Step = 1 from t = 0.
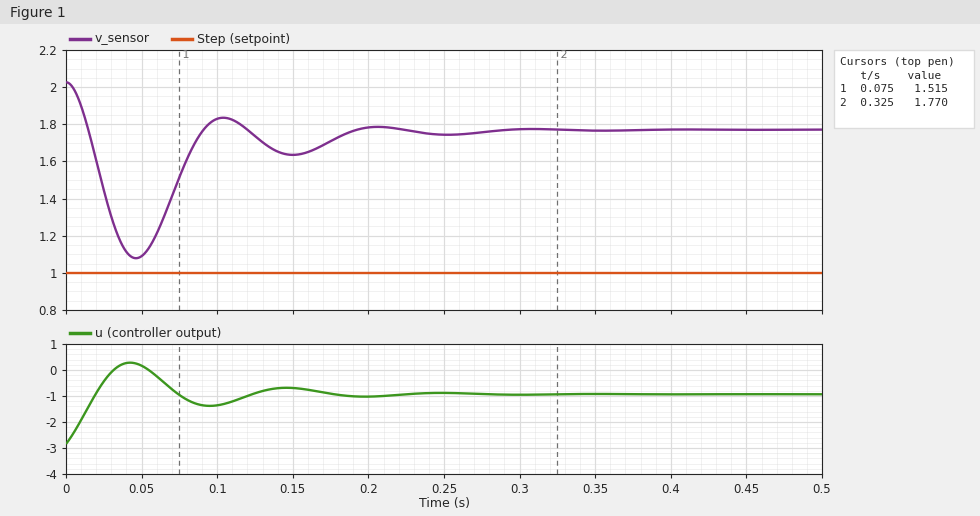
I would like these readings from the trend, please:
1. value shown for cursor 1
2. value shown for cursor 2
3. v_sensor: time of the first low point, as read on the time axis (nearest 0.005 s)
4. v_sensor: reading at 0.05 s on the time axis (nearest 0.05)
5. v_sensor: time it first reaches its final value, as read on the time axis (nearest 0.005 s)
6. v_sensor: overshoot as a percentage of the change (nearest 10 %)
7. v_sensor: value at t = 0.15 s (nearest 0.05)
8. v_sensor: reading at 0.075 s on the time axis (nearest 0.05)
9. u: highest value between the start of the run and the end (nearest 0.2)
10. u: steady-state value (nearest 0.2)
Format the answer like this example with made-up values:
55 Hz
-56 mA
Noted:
1.515
1.770
0.045 s
1.10
0.015 s
270 %
1.65
1.50
0.2
-1.0
